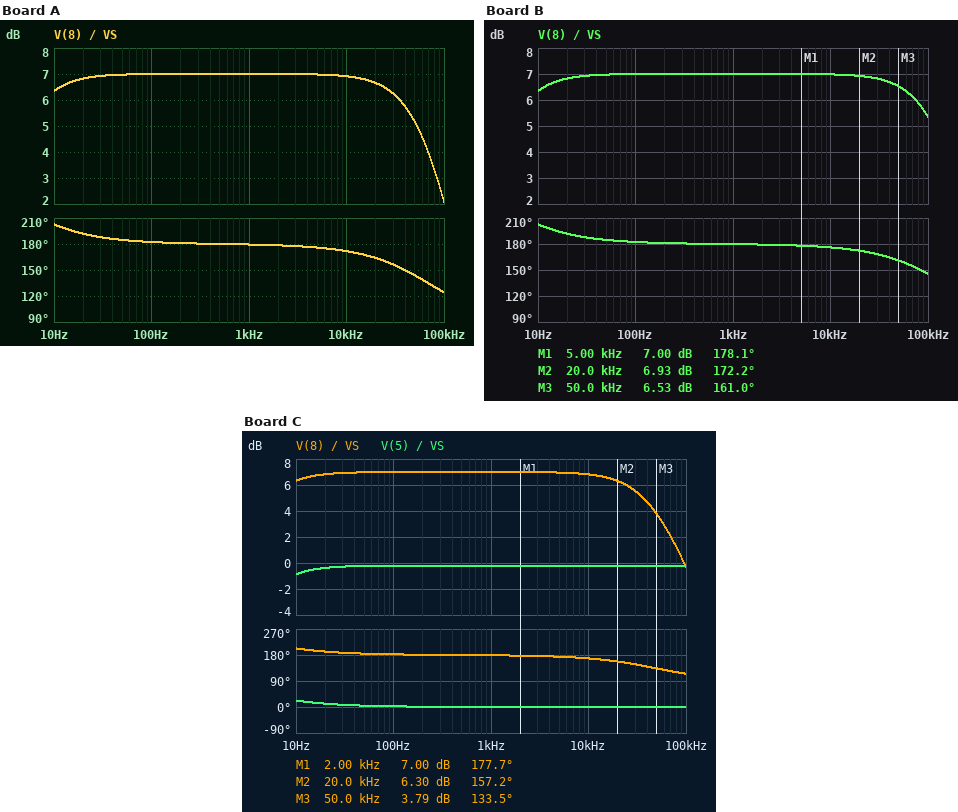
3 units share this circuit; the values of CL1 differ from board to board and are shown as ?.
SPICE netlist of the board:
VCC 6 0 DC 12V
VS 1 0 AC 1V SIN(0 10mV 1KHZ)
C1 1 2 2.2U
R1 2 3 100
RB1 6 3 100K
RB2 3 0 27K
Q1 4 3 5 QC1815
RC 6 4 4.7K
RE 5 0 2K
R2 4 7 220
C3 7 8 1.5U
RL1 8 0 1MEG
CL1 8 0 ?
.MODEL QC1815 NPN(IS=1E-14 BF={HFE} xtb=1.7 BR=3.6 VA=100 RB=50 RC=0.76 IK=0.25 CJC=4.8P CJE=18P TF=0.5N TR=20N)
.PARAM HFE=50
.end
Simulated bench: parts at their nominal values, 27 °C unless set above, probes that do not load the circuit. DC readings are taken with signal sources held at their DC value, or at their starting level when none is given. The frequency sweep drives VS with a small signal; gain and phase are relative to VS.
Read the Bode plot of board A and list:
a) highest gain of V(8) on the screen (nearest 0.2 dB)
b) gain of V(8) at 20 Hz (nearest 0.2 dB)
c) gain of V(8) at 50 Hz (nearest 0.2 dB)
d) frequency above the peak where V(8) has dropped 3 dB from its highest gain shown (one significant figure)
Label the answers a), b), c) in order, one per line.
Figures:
a) 7.0 dB
b) 6.8 dB
c) 7.0 dB
d) 70 kHz
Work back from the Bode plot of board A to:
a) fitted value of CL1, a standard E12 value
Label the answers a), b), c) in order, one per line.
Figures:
a) 470 pF
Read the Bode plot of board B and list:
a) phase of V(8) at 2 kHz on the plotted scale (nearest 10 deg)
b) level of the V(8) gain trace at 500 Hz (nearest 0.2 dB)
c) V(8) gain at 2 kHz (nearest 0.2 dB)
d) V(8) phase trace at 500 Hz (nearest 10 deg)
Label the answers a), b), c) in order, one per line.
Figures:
a) 180 deg
b) 7.0 dB
c) 7.0 dB
d) 180 deg
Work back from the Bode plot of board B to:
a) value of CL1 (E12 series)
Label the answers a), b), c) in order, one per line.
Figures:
a) 220 pF
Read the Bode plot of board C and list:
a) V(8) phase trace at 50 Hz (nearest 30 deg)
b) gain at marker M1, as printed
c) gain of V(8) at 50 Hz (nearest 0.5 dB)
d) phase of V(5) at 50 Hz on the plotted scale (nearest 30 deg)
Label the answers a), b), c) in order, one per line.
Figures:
a) 180 deg
b) 7.00 dB
c) 7.0 dB
d) 0 deg
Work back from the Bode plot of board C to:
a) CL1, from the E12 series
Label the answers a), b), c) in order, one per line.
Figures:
a) 680 pF
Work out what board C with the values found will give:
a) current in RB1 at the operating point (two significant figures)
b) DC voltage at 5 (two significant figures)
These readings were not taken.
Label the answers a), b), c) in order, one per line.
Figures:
a) 98 µA
b) 1.6 V
